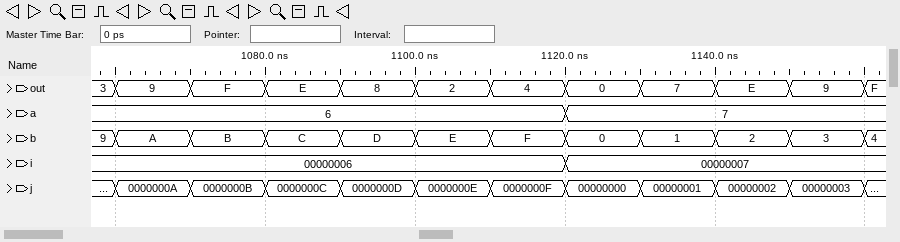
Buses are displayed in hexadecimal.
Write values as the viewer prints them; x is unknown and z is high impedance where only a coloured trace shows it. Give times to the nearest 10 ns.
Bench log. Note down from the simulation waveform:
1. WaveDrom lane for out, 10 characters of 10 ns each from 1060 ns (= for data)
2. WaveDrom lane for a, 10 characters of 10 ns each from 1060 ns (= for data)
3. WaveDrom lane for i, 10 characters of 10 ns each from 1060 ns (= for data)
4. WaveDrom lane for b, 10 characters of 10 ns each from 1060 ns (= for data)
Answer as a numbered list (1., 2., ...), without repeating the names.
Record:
1. {name: 'out', wave: '==========', data: '9 F E 8 2 4 0 7 E 9'}
2. {name: 'a', wave: '=.....=...', data: '6 7'}
3. {name: 'i', wave: '=.....=...', data: '00000006 00000007'}
4. {name: 'b', wave: '==========', data: 'A B C D E F 0 1 2 3'}
